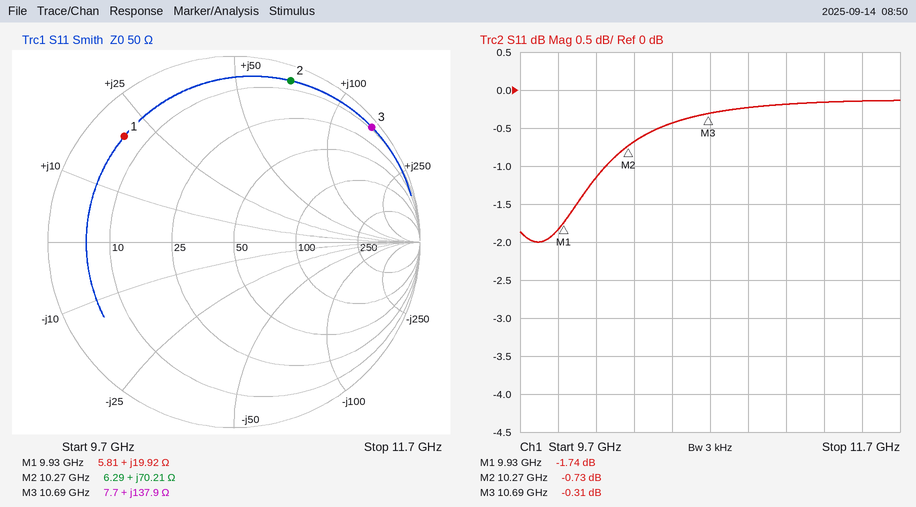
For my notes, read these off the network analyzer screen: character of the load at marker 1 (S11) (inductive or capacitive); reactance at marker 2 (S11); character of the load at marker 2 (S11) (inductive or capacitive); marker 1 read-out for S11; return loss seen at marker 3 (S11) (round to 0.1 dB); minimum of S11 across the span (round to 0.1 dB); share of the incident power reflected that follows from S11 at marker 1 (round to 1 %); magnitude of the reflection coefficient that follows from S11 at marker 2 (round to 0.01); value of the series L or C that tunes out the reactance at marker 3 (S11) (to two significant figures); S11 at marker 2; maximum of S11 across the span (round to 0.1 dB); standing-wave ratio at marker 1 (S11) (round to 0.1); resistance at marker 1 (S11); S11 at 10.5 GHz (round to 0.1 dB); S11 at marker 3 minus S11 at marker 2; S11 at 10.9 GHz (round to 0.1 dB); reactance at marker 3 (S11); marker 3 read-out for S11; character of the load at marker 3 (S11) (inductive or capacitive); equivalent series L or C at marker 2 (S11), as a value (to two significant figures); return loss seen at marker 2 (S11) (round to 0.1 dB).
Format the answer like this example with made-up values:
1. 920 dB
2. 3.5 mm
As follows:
1. inductive
2. +70.21 Ω
3. inductive
4. -1.74 dB
5. 0.3 dB
6. -2.0 dB
7. 67 %
8. 0.92
9. 110 fF
10. -0.73 dB
11. -0.1 dB
12. 10.0
13. 5.81 Ω
14. -0.4 dB
15. 0.42 dB
16. -0.2 dB
17. +137.9 Ω
18. -0.31 dB
19. inductive
20. 1.1 nH
21. 0.7 dB
